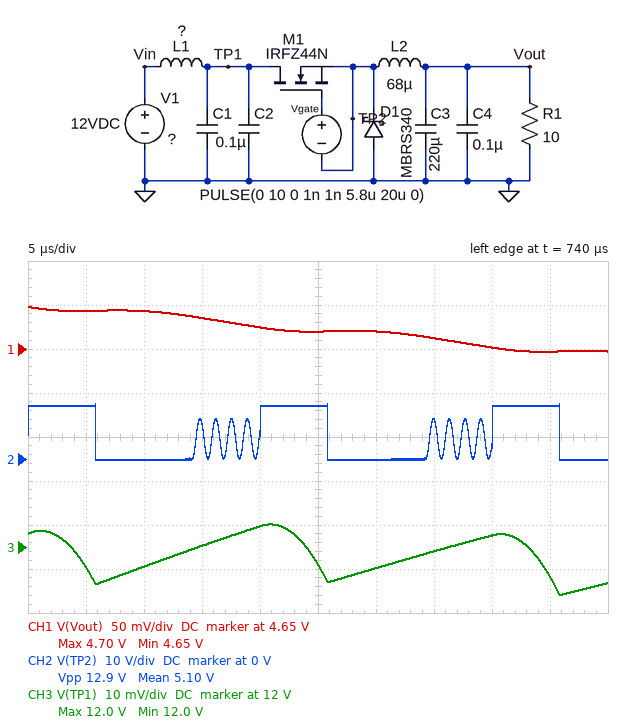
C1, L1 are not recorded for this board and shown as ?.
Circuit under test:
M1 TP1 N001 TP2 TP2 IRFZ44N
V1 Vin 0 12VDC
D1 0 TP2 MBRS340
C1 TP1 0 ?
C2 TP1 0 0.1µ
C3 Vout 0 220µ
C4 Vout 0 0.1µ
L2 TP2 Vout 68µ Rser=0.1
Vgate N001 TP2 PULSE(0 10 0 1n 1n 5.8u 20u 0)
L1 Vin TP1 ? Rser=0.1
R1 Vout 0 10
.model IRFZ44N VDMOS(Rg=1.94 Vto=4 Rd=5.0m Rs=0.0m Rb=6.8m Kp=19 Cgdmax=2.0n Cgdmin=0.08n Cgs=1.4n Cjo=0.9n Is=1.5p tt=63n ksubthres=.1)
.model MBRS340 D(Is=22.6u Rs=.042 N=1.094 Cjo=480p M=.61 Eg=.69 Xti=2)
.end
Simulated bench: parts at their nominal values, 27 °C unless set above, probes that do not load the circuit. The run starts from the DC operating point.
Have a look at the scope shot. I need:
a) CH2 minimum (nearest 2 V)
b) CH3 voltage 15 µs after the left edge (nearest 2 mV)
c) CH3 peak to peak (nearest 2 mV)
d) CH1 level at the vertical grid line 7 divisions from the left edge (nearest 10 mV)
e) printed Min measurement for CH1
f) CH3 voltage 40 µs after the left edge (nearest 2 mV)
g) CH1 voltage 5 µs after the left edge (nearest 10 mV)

0 V
12.000 V
16 mV
4.66 V
4.65 V
12.002 V
4.69 V
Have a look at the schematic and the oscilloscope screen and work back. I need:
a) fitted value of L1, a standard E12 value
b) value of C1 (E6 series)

8.2 µH
100 µF
